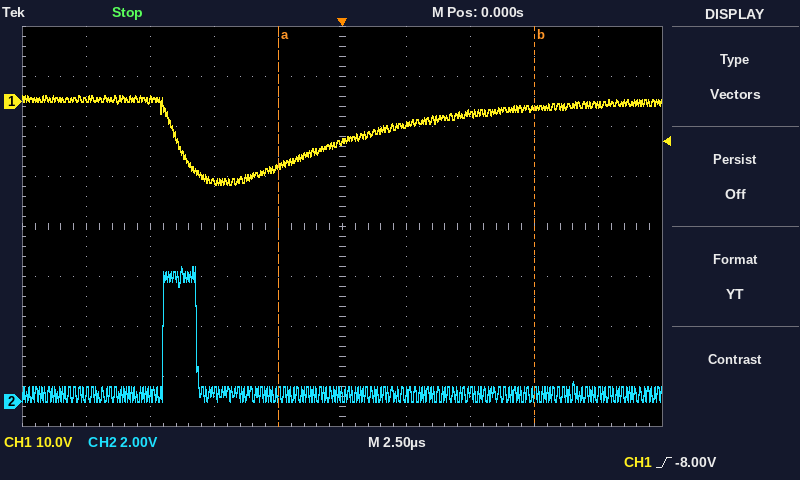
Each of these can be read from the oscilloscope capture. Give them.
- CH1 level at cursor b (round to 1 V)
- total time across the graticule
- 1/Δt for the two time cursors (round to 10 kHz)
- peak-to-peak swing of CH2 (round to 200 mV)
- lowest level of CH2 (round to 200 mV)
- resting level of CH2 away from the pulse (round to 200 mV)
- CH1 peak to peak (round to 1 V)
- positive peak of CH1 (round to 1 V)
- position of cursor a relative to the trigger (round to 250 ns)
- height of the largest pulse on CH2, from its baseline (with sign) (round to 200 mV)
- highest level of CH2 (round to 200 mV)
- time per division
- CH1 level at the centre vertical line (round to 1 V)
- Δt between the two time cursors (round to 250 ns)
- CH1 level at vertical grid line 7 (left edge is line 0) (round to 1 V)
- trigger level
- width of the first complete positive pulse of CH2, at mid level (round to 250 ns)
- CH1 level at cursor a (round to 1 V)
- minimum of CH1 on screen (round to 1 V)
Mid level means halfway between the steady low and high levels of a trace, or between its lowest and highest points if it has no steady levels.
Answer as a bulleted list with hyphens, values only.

- -1 V
- 25 µs
- 100 kHz
- 5.4 V
- 0.0 V
- 400 mV
- 18 V
- 1 V
- -2.50 µs
- +5.0 V
- 5.4 V
- 2.5 µs
- -8 V
- 10.00 µs
- -2 V
- -8.00 V
- 1.25 µs
- -13 V
- -17 V
